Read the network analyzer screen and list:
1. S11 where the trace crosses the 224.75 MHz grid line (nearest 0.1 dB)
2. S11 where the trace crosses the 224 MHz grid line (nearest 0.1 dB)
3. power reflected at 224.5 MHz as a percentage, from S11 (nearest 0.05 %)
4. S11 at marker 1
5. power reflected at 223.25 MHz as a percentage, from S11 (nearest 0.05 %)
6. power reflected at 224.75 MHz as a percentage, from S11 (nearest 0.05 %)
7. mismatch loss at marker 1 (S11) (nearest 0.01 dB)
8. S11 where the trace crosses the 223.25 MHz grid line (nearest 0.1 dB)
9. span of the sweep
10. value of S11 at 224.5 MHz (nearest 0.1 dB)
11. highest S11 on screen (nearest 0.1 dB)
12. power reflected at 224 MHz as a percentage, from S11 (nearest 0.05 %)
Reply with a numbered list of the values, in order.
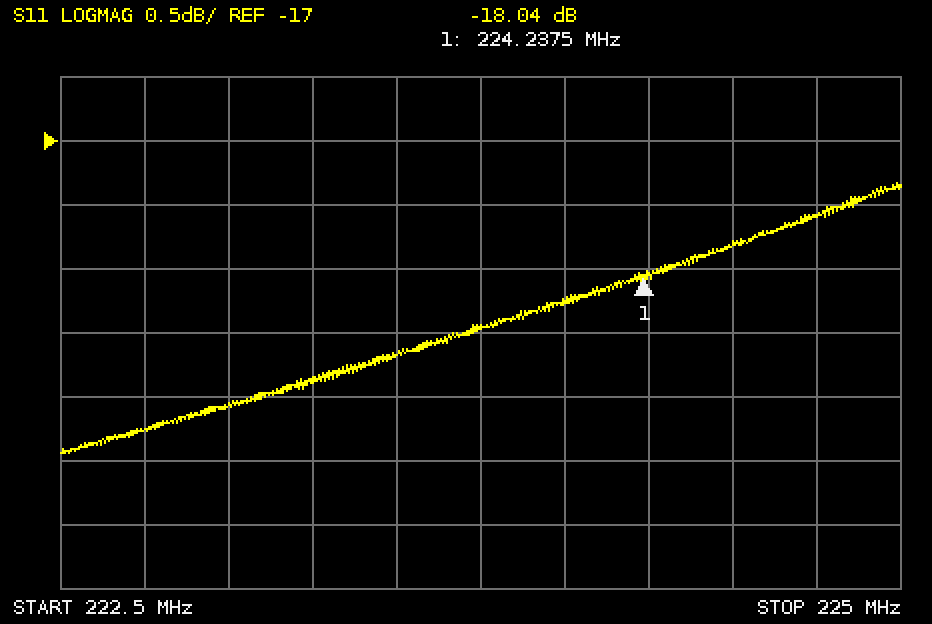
1. -17.6 dB
2. -18.3 dB
3. 1.65 %
4. -18.04 dB
5. 1.30 %
6. 1.75 %
7. 0.07 dB
8. -18.9 dB
9. 2.5 MHz
10. -17.8 dB
11. -17.3 dB
12. 1.50 %
